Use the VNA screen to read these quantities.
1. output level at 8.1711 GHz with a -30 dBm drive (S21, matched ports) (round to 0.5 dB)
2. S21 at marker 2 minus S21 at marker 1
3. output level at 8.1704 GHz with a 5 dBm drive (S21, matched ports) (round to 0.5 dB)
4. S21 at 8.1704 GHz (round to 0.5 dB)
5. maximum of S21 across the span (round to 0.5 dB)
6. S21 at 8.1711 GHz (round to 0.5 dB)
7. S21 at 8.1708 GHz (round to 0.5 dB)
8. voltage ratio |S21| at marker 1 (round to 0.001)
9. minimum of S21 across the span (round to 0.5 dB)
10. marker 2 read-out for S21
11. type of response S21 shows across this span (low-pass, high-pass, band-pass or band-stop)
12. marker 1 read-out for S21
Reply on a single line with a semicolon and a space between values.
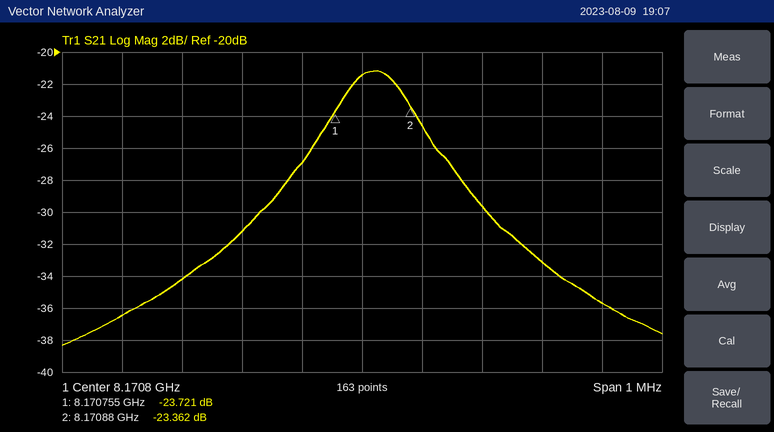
-63.0 dBm; 0.359 dB; -31.5 dBm; -36.5 dB; -21.0 dB; -33.0 dB; -21.5 dB; 0.065; -38.5 dB; -23.362 dB; band-pass; -23.721 dB
